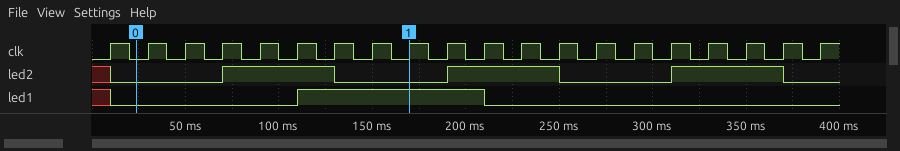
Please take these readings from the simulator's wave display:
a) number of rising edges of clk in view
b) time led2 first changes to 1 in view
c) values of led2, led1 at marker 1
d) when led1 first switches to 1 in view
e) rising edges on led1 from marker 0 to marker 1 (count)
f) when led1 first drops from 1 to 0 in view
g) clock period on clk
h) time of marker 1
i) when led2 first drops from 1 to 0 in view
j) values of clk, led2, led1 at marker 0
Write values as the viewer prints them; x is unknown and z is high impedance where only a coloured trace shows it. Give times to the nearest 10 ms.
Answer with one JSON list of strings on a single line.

["20", "70 ms", "led2=0, led1=1", "110 ms", "1", "210 ms", "20 ms", "170 ms", "130 ms", "clk=0, led2=0, led1=0"]
